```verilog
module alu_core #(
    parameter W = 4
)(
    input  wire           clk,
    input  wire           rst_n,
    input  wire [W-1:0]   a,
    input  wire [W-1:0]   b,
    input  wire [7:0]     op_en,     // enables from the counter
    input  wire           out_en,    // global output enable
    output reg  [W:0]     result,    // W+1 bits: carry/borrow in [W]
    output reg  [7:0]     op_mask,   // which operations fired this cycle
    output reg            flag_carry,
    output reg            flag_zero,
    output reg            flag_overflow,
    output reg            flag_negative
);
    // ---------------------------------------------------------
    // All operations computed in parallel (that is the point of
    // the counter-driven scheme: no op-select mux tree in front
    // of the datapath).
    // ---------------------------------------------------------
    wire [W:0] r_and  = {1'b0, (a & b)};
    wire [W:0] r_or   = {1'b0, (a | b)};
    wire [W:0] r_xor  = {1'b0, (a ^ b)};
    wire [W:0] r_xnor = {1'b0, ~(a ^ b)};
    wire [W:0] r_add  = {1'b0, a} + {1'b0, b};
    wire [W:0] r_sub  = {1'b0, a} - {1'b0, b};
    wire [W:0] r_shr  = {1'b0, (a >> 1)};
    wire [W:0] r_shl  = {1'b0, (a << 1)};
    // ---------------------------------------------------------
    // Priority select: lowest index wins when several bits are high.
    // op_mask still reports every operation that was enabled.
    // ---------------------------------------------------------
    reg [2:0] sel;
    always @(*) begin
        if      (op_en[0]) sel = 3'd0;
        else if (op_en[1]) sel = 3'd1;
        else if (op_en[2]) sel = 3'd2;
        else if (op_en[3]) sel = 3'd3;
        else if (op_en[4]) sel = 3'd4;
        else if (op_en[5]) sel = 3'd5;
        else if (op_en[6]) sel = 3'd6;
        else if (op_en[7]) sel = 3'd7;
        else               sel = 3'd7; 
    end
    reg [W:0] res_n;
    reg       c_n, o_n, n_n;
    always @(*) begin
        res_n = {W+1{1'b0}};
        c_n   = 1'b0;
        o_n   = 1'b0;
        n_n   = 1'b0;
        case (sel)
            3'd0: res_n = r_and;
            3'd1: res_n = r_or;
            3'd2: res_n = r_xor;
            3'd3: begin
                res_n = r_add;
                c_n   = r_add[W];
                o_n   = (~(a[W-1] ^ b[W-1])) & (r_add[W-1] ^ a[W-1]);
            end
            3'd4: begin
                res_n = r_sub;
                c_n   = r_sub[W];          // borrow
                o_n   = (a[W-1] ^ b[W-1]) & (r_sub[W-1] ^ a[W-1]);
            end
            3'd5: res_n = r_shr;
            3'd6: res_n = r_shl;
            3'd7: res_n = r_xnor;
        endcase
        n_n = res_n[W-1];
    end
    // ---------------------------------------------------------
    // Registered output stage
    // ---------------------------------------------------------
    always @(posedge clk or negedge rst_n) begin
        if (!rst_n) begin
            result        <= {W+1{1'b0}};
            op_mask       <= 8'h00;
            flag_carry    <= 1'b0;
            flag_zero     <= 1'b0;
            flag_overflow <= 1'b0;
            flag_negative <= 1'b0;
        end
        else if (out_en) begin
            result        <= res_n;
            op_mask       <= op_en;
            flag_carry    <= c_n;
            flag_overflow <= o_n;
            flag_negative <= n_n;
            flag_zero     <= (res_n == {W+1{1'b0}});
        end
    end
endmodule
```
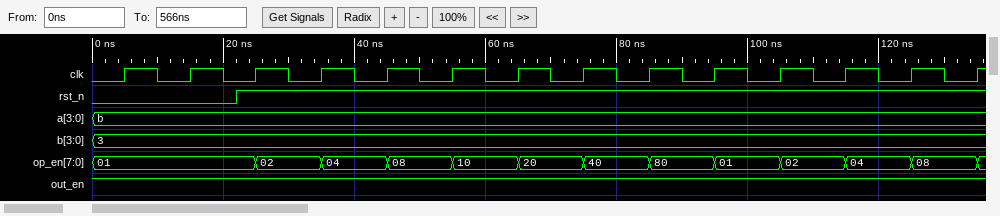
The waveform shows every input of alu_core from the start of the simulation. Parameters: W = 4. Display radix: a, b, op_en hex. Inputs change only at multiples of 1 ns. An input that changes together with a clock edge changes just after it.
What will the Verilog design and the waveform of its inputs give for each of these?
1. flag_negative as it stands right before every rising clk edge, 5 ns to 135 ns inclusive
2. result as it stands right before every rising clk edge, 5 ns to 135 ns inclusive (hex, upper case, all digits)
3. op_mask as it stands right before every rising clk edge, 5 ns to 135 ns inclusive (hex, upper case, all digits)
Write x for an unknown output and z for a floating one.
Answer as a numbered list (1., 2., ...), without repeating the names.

1. 0 0 0 0 1 1 1 1 0 0 0 0 1 1
2. 00, 00, 00, 03, 0B, 08, 0E, 08, 05, 06, 07, 03, 0B, 08
3. 00, 00, 00, 01, 02, 04, 08, 10, 20, 40, 80, 01, 02, 04
